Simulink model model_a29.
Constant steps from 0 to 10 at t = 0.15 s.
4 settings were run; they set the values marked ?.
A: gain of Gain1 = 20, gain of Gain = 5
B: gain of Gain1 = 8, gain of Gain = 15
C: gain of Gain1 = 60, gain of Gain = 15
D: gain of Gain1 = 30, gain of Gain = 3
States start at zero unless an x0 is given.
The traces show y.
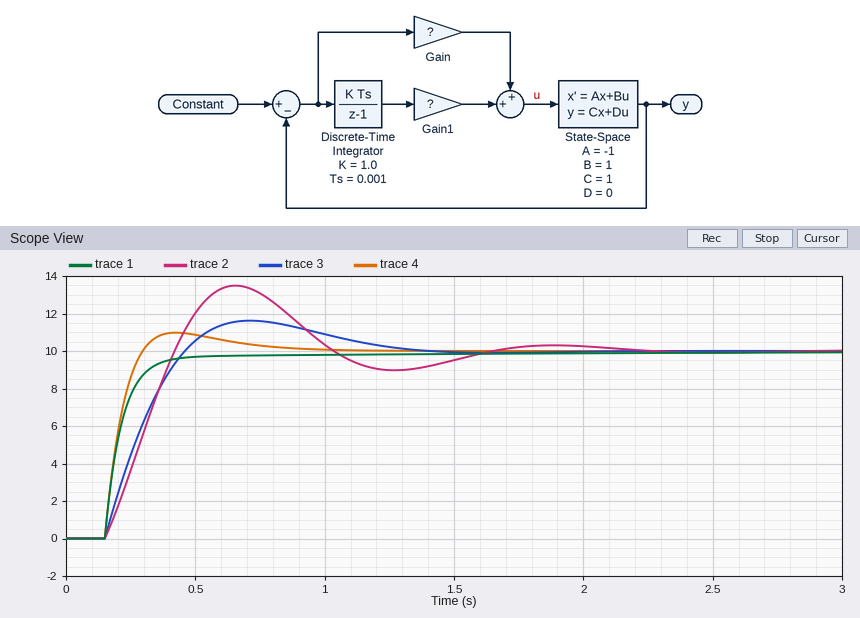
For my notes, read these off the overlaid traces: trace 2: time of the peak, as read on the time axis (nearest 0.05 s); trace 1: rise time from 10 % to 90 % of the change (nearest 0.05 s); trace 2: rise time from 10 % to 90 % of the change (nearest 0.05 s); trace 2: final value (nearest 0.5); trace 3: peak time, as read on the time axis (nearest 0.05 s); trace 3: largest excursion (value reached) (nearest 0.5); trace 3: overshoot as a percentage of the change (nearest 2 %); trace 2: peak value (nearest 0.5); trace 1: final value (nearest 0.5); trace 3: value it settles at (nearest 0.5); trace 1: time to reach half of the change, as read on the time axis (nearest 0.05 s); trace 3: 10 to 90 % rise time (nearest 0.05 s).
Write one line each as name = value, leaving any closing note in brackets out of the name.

trace 2: time of the peak, as read on the time axis = 0.65 s
trace 1: rise time from 10 % to 90 % of the change = 0.15 s
trace 2: rise time from 10 % to 90 % of the change = 0.20 s
trace 2: final value = 10.0
trace 3: peak time, as read on the time axis = 0.70 s
trace 3: largest excursion (value reached) = 11.5
trace 3: overshoot as a percentage of the change = 16 %
trace 2: peak value = 13.5
trace 1: final value = 10.0
trace 3: value it settles at = 10.0
trace 1: time to reach half of the change, as read on the time axis = 0.20 s
trace 3: 10 to 90 % rise time = 0.25 s
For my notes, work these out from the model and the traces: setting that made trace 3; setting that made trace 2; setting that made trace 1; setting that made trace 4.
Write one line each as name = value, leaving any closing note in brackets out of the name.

setting that made trace 3 = A
setting that made trace 2 = D
setting that made trace 1 = B
setting that made trace 4 = C
